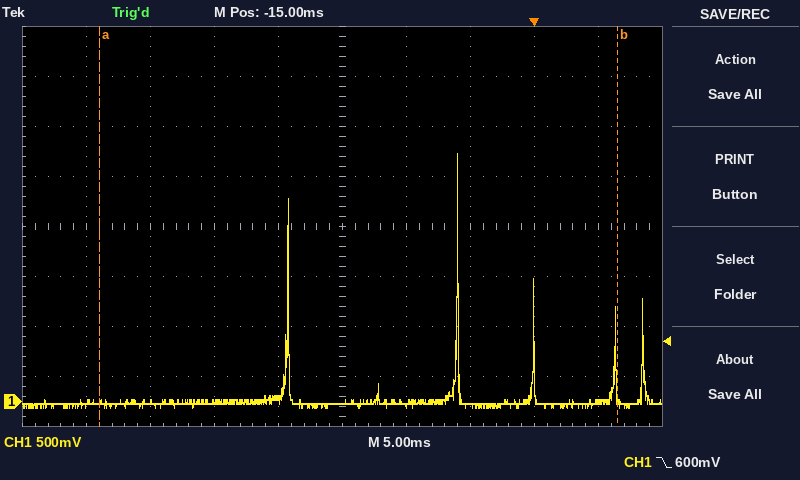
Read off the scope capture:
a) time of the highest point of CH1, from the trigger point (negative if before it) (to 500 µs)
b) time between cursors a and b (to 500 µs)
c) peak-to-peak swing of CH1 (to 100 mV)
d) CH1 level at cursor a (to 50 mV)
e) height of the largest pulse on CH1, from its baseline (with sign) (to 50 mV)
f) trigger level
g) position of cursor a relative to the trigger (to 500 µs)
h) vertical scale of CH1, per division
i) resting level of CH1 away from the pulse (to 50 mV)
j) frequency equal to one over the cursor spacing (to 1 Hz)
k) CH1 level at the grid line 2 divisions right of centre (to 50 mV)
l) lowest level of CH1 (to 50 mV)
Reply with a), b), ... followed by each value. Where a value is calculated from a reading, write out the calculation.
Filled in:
a) -6.0 ms
b) 40.5 ms
c) 2.50 V
d) 0 mV
e) +2.50 V
f) 600 mV
g) -34.0 ms
h) 500 mV
i) 0 mV
j) 1 / 40.5 ms ≈ 25 Hz
k) -50 mV
l) -50 mV
